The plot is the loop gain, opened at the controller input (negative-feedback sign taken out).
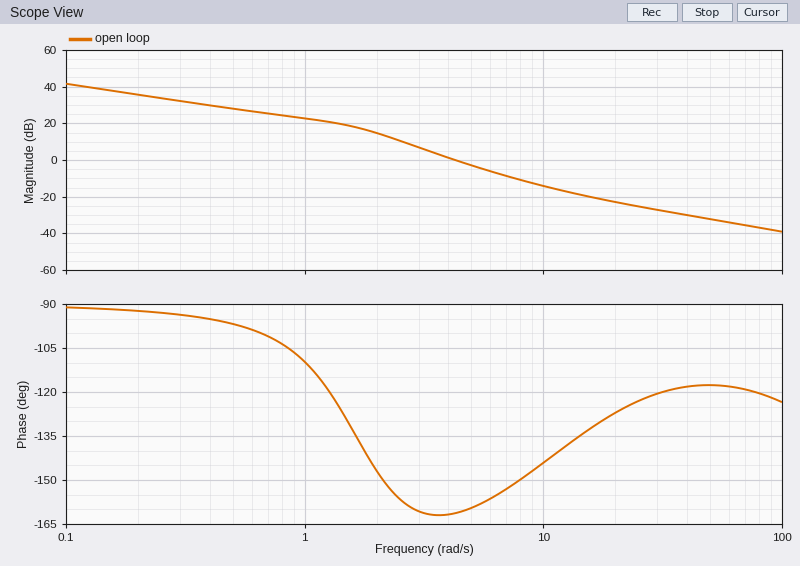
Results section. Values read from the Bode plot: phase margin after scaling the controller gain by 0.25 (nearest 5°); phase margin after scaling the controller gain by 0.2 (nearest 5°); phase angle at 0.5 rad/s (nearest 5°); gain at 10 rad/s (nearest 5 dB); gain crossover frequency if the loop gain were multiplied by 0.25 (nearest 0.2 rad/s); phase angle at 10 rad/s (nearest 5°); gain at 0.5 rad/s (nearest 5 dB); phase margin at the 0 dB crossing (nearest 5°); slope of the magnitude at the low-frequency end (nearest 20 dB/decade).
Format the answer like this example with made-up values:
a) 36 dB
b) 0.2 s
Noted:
a) 25°
b) 30°
c) -95°
d) -15 dB
e) 2.4 rad/s
f) -145°
g) 30 dB
h) 20°
i) -20 dB/decade
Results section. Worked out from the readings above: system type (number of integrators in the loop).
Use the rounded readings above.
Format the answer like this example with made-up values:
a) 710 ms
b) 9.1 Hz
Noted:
a) 1
